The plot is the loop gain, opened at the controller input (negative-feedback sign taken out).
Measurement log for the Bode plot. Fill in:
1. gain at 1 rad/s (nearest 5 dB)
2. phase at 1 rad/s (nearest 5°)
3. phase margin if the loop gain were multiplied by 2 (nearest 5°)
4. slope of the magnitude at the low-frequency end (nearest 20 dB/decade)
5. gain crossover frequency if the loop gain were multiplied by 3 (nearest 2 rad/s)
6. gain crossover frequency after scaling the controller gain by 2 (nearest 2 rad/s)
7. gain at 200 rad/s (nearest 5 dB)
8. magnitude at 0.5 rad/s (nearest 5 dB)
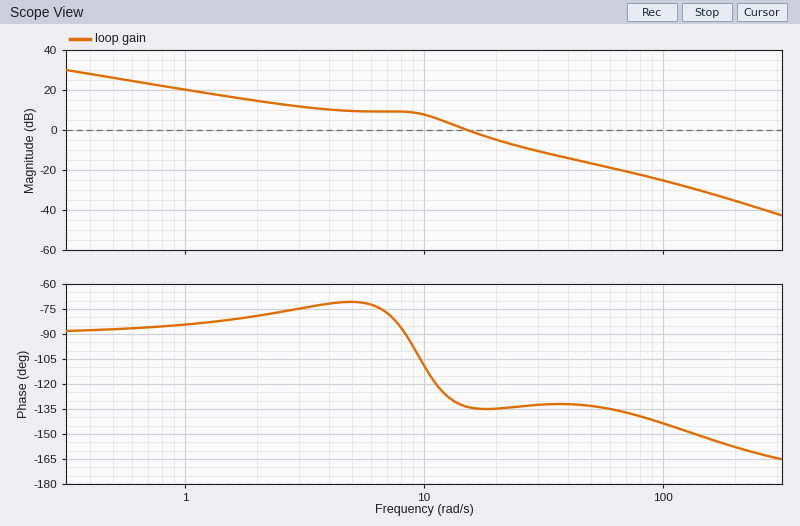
20 dB
-85°
45°
-20 dB/decade
28 rad/s
22 rad/s
-35 dB
25 dB
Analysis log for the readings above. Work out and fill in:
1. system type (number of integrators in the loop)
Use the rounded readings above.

1
